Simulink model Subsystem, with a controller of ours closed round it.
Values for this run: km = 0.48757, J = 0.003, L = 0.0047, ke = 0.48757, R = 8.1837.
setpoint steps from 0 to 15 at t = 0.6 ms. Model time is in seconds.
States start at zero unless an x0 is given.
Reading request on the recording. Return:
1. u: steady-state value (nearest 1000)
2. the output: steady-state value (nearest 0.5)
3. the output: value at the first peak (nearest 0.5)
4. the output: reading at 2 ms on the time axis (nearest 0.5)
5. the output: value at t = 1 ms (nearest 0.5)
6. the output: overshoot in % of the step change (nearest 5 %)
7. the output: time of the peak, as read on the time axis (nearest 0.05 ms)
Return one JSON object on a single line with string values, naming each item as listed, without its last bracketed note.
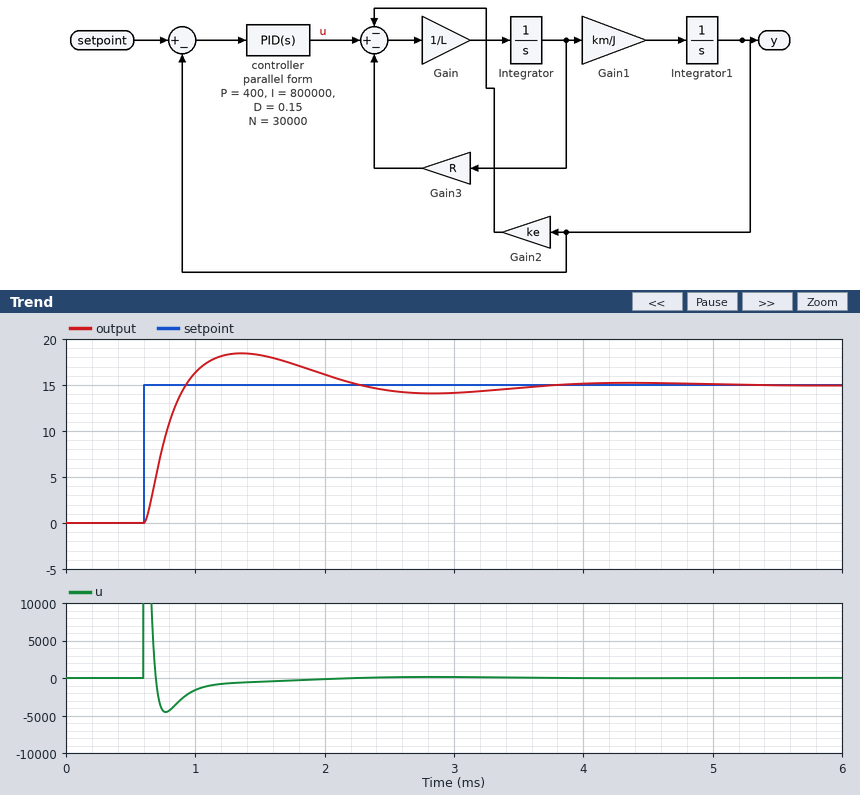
{"u: steady-state value": "0", "the output: steady-state value": "15.0", "the output: value at the first peak": "18.5", "the output: reading at 2 ms on the time axis": "16.0", "the output: value at t = 1 ms": "16.5", "the output: overshoot in % of the step change": "25 %", "the output: time of the peak, as read on the time axis": "1.35 ms"}
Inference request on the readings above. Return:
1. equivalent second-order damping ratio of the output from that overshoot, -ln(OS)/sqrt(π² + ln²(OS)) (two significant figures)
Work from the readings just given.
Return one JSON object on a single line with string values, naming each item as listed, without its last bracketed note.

{"equivalent second-order damping ratio of the output from that overshoot, -ln(OS)/sqrt(π² + ln²(OS))": "0.40"}
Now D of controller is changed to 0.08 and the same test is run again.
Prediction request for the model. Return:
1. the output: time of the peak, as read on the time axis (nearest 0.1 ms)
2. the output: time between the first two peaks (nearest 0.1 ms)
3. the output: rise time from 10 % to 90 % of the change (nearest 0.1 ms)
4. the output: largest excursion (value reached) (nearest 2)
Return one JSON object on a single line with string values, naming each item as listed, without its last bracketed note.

{"the output: time of the peak, as read on the time axis": "1.4 ms", "the output: time between the first two peaks": "2.1 ms", "the output: rise time from 10 % to 90 % of the change": "0.3 ms", "the output: largest excursion (value reached)": "22"}
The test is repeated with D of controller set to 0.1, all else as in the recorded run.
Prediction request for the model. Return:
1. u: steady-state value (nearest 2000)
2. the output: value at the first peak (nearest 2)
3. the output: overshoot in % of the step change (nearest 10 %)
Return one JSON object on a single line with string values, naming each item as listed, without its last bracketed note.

{"u: steady-state value": "0", "the output: value at the first peak": "20", "the output: overshoot in % of the step change": "40 %"}
